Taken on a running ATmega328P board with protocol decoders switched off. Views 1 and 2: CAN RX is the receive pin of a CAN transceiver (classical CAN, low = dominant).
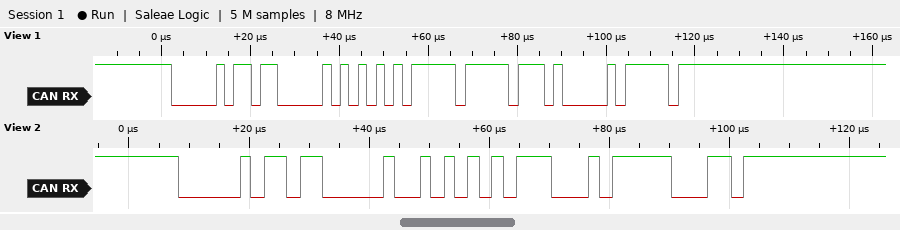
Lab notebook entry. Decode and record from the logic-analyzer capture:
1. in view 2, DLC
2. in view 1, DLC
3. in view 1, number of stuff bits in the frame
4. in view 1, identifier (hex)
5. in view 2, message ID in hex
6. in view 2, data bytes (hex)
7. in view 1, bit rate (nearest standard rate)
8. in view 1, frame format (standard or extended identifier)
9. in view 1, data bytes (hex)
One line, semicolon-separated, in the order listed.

1; 2; 5; 0x036; 0x036; 55; 500 kbit/s; standard; AB FF
